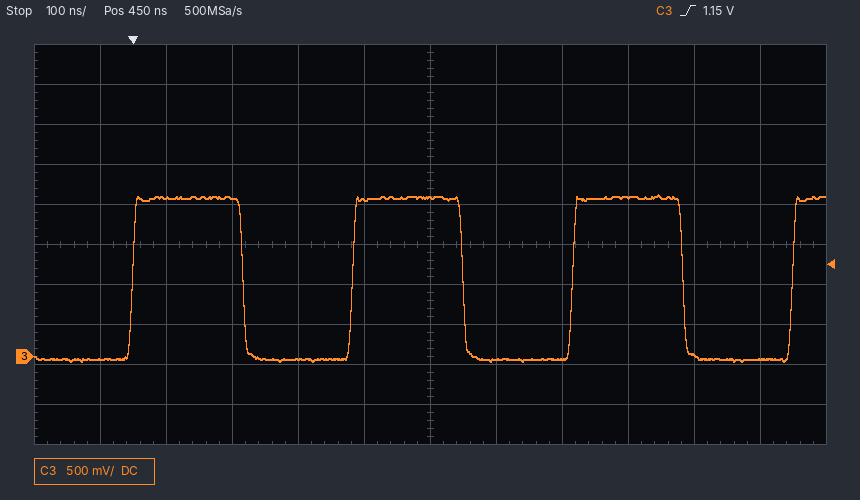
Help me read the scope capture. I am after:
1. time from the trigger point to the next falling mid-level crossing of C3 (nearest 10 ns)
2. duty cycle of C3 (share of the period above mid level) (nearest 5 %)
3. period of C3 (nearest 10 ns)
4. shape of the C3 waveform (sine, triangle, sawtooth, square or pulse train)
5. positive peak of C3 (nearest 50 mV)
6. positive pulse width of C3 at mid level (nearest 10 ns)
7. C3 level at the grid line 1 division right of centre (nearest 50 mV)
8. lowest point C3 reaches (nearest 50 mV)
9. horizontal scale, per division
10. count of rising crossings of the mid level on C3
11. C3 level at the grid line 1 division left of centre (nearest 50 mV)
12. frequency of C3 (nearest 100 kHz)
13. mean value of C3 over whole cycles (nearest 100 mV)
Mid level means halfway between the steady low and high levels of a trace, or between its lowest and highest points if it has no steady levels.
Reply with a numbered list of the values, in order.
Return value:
1. 170 ns
2. 50 %
3. 330 ns
4. square
5. 2.00 V
6. 170 ns
7. -50 mV
8. -50 mV
9. 100 ns
10. 4
11. 1.95 V
12. 3.0 MHz
13. 1.0 V
